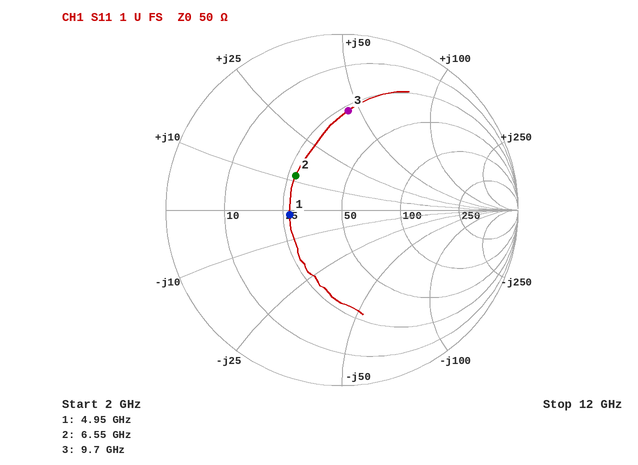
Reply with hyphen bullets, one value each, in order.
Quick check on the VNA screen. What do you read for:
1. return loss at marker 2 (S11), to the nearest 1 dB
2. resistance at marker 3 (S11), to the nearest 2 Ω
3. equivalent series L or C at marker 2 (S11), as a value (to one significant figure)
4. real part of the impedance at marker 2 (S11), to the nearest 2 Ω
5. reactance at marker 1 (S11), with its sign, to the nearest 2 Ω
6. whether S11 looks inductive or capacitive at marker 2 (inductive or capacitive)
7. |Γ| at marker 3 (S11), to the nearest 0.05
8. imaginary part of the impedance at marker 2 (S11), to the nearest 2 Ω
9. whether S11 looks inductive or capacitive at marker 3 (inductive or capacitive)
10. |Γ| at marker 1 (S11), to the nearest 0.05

- 10 dB
- 28 Ω
- 300 pH
- 28 Ω
- -2 Ω
- inductive
- 0.55
- +12 Ω
- inductive
- 0.30
